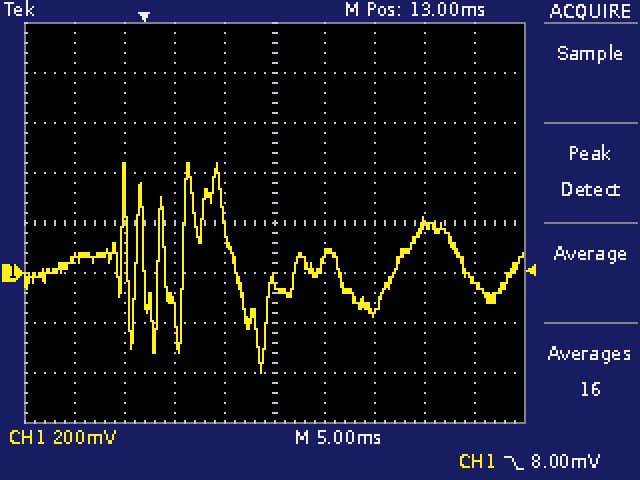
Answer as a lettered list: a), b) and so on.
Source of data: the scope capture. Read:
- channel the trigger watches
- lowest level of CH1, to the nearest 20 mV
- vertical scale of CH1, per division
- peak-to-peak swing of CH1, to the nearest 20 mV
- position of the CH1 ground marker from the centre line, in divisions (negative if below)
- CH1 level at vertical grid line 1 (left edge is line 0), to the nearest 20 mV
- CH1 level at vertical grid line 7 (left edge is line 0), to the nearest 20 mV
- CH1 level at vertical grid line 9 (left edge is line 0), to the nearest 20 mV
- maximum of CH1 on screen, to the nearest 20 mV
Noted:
a) CH1
b) -400 mV
c) 200 mV
d) 840 mV
e) -1.0 div
f) 60 mV
g) -160 mV
h) -40 mV
i) 440 mV
